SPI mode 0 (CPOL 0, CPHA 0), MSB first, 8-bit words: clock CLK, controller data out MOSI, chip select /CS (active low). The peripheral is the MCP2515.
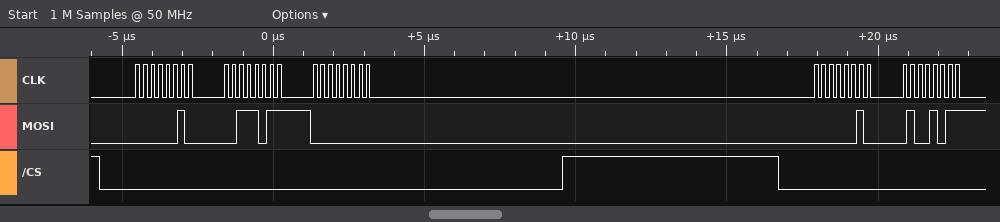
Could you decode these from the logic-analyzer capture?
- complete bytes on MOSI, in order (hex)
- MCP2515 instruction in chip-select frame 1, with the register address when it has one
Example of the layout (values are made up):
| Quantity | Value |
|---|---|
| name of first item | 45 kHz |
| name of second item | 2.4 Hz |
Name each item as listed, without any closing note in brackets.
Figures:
| Quantity | Value |
|---|---|
| complete bytes on MOSI, in order | 02 3B 00 02 4B |
| MCP2515 instruction in chip-select frame 1, with the register address when it has one | WRITE 0x3B |
